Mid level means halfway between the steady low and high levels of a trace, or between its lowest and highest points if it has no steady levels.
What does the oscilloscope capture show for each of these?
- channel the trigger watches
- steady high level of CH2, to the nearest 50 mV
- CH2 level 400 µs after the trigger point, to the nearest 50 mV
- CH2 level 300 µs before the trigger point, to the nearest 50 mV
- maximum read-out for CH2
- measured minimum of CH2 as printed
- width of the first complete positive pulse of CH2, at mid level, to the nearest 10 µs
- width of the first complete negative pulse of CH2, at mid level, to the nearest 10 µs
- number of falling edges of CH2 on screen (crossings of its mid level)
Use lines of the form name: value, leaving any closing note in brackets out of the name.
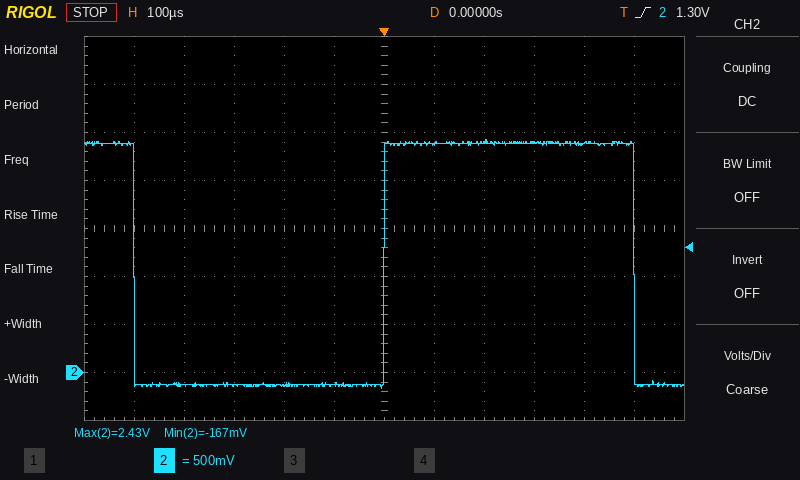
channel the trigger watches: CH2
steady high level of CH2, to the nearest 50 mV: 2.40 V
CH2 level 400 µs after the trigger point, to the nearest 50 mV: 2.40 V
CH2 level 300 µs before the trigger point, to the nearest 50 mV: -150 mV
maximum read-out for CH2: 2.43 V
measured minimum of CH2 as printed: -167 mV
width of the first complete positive pulse of CH2, at mid level, to the nearest 10 µs: 500 µs
width of the first complete negative pulse of CH2, at mid level, to the nearest 10 µs: 500 µs
number of falling edges of CH2 on screen: 2
